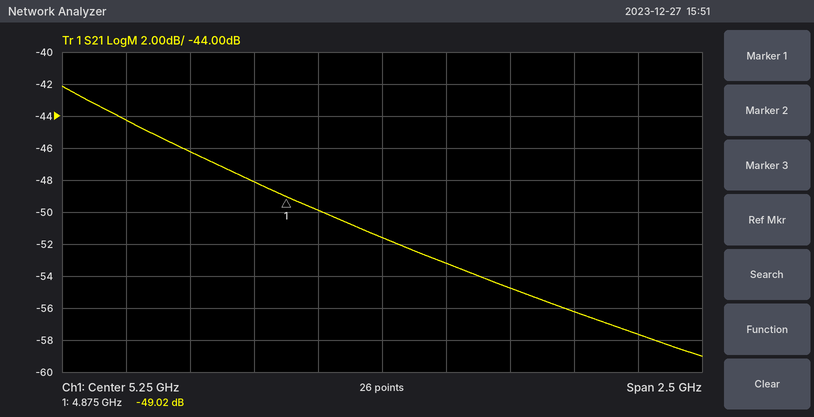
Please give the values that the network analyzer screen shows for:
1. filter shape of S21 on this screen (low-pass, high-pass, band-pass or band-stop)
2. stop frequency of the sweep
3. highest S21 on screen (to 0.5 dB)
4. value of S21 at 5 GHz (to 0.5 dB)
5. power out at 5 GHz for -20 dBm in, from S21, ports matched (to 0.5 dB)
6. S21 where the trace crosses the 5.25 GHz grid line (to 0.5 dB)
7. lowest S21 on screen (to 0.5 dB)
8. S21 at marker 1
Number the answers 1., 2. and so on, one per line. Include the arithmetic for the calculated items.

1. low-pass
2. 6.5 GHz
3. -42.0 dB
4. -50.0 dB
5. -20 dBm + (-50.0 dB) = -70.0 dBm
6. -51.5 dB
7. -59.0 dB
8. -49.02 dB
